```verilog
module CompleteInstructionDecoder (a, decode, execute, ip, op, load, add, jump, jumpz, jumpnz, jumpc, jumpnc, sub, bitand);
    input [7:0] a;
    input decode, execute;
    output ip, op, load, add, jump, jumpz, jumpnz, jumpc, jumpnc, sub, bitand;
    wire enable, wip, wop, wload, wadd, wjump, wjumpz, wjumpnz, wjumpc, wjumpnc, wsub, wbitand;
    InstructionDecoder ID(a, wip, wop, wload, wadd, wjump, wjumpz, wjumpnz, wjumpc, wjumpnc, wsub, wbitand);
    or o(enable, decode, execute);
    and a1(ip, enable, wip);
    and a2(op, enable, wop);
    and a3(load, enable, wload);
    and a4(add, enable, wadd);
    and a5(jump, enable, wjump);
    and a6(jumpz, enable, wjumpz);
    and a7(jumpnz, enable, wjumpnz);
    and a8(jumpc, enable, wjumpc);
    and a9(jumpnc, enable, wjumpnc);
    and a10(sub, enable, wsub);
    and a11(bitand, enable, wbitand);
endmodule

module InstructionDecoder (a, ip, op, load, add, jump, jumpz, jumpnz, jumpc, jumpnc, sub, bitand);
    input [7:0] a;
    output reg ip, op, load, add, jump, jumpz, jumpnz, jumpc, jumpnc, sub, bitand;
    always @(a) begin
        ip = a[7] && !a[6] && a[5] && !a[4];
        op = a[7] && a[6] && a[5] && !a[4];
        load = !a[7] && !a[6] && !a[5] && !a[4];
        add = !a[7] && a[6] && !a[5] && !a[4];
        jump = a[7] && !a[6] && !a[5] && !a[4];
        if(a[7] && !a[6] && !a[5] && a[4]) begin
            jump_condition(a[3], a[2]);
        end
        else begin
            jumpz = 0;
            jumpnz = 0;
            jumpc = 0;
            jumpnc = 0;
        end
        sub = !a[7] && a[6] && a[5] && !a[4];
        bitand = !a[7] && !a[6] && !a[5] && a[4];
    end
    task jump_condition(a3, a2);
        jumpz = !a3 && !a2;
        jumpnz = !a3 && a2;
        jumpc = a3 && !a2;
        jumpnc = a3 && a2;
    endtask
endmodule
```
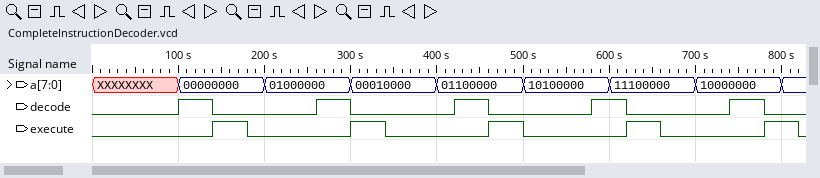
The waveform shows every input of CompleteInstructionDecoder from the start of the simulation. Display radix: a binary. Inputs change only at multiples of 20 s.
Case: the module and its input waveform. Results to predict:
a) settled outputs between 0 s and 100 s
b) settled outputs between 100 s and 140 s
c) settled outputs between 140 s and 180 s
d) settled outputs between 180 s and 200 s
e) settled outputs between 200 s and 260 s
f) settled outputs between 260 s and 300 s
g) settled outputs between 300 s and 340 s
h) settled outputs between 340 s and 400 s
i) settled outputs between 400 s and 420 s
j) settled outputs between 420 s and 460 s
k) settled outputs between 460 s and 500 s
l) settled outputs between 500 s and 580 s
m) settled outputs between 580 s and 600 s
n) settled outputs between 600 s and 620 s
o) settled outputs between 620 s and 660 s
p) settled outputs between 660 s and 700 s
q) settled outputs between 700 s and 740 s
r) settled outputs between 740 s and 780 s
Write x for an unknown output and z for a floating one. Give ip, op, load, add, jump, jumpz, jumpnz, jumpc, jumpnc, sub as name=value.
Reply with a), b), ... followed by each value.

a) ip=0, op=0, load=0, add=0, jump=0, jumpz=0, jumpnz=0, jumpc=0, jumpnc=0, sub=0
b) ip=0, op=0, load=1, add=0, jump=0, jumpz=0, jumpnz=0, jumpc=0, jumpnc=0, sub=0
c) ip=0, op=0, load=1, add=0, jump=0, jumpz=0, jumpnz=0, jumpc=0, jumpnc=0, sub=0
d) ip=0, op=0, load=0, add=0, jump=0, jumpz=0, jumpnz=0, jumpc=0, jumpnc=0, sub=0
e) ip=0, op=0, load=0, add=0, jump=0, jumpz=0, jumpnz=0, jumpc=0, jumpnc=0, sub=0
f) ip=0, op=0, load=0, add=1, jump=0, jumpz=0, jumpnz=0, jumpc=0, jumpnc=0, sub=0
g) ip=0, op=0, load=0, add=0, jump=0, jumpz=0, jumpnz=0, jumpc=0, jumpnc=0, sub=0
h) ip=0, op=0, load=0, add=0, jump=0, jumpz=0, jumpnz=0, jumpc=0, jumpnc=0, sub=0
i) ip=0, op=0, load=0, add=0, jump=0, jumpz=0, jumpnz=0, jumpc=0, jumpnc=0, sub=0
j) ip=0, op=0, load=0, add=0, jump=0, jumpz=0, jumpnz=0, jumpc=0, jumpnc=0, sub=1
k) ip=0, op=0, load=0, add=0, jump=0, jumpz=0, jumpnz=0, jumpc=0, jumpnc=0, sub=1
l) ip=0, op=0, load=0, add=0, jump=0, jumpz=0, jumpnz=0, jumpc=0, jumpnc=0, sub=0
m) ip=1, op=0, load=0, add=0, jump=0, jumpz=0, jumpnz=0, jumpc=0, jumpnc=0, sub=0
n) ip=0, op=1, load=0, add=0, jump=0, jumpz=0, jumpnz=0, jumpc=0, jumpnc=0, sub=0
o) ip=0, op=1, load=0, add=0, jump=0, jumpz=0, jumpnz=0, jumpc=0, jumpnc=0, sub=0
p) ip=0, op=0, load=0, add=0, jump=0, jumpz=0, jumpnz=0, jumpc=0, jumpnc=0, sub=0
q) ip=0, op=0, load=0, add=0, jump=0, jumpz=0, jumpnz=0, jumpc=0, jumpnc=0, sub=0
r) ip=0, op=0, load=0, add=0, jump=1, jumpz=0, jumpnz=0, jumpc=0, jumpnc=0, sub=0
